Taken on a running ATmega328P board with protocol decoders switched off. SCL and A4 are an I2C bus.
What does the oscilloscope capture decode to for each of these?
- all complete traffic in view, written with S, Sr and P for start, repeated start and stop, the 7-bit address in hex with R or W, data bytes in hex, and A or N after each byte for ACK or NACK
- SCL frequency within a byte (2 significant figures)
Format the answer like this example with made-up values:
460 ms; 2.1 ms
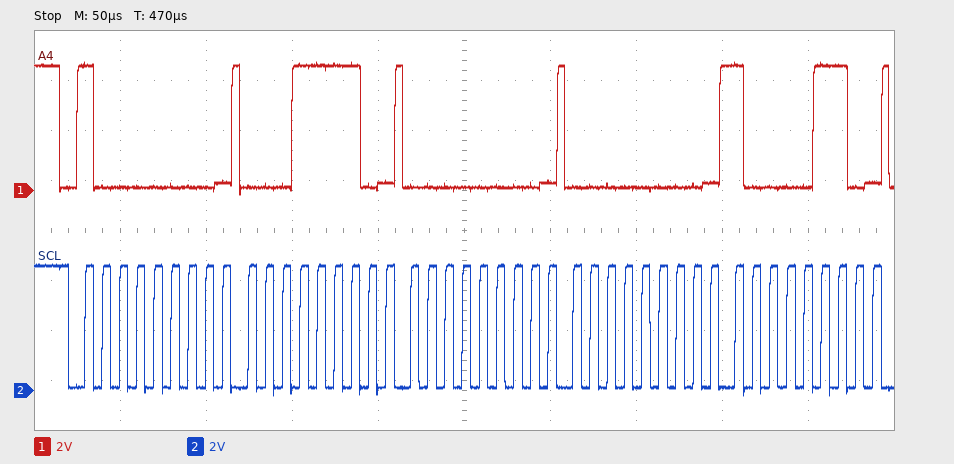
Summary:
S 40W A 1E A 00 A 00 A 86 A; 100 kHz
